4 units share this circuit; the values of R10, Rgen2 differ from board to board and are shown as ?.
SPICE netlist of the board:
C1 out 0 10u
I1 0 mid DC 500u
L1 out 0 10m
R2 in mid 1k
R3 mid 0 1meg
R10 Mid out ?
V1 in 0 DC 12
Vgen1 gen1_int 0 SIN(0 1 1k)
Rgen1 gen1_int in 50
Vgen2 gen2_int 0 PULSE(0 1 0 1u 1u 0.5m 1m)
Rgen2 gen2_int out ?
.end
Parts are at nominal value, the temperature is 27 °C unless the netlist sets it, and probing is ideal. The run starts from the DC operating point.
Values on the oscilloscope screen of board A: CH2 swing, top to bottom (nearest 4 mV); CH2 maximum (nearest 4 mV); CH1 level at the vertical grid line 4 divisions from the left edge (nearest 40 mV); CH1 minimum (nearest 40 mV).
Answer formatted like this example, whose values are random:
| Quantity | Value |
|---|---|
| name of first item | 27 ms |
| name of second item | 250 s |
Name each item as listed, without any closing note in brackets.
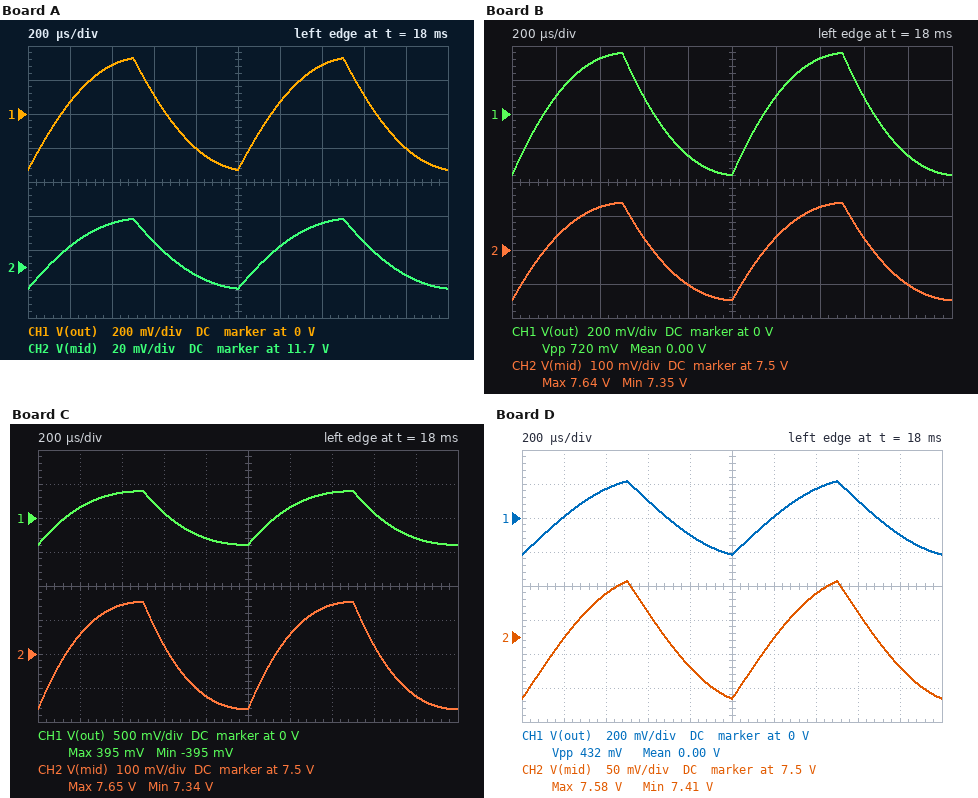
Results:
| Quantity | Value |
|---|---|
| CH2 swing, top to bottom | 40 mV |
| CH2 maximum | 11.728 V |
| CH1 level at the vertical grid line 4 divisions from the left edge | -200 mV |
| CH1 minimum | -320 mV |
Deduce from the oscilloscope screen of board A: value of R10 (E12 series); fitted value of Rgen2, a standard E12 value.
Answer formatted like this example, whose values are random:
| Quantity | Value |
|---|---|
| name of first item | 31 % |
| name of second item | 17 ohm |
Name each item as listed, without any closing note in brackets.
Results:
| Quantity | Value |
|---|---|
| value of R10 | 15 kΩ |
| fitted value of Rgen2, a standard E12 value | 39 Ω |
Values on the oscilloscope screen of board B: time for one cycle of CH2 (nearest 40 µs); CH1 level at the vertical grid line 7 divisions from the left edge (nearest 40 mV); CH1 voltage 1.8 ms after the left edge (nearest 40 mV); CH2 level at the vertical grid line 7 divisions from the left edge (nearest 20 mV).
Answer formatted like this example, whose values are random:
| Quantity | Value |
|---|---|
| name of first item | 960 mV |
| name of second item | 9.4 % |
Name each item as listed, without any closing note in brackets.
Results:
| Quantity | Value |
|---|---|
| time for one cycle of CH2 | 1.00 ms |
| CH1 level at the vertical grid line 7 divisions from the left edge | 320 mV |
| CH1 voltage 1.8 ms after the left edge | -240 mV |
| CH2 level at the vertical grid line 7 divisions from the left edge | 7.62 V |
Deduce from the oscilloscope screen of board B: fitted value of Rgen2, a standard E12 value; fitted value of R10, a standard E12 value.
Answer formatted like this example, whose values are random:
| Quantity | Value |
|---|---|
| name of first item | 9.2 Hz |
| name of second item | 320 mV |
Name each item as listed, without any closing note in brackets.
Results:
| Quantity | Value |
|---|---|
| fitted value of Rgen2, a standard E12 value | 33 Ω |
| fitted value of R10, a standard E12 value | 1.5 kΩ |
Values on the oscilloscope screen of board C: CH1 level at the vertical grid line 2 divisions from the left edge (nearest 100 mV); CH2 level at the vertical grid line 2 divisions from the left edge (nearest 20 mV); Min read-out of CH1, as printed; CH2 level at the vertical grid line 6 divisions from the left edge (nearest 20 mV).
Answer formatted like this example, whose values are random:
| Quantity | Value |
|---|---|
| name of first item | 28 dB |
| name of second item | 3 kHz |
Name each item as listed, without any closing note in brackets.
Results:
| Quantity | Value |
|---|---|
| CH1 level at the vertical grid line 2 divisions from the left edge | 400 mV |
| CH2 level at the vertical grid line 2 divisions from the left edge | 7.64 V |
| Min read-out of CH1, as printed | -395 mV |
| CH2 level at the vertical grid line 6 divisions from the left edge | 7.56 V |
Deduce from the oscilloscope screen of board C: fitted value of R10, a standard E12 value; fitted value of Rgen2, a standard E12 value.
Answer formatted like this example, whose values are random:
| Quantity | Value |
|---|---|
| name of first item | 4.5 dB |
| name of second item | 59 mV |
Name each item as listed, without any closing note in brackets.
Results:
| Quantity | Value |
|---|---|
| fitted value of R10, a standard E12 value | 1.5 kΩ |
| fitted value of Rgen2, a standard E12 value | 27 Ω |
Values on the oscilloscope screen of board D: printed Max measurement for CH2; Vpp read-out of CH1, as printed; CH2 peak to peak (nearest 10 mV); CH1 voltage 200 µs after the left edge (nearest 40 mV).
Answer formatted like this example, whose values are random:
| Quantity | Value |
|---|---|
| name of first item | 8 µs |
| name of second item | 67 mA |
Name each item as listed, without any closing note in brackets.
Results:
| Quantity | Value |
|---|---|
| printed Max measurement for CH2 | 7.58 V |
| Vpp read-out of CH1, as printed | 432 mV |
| CH2 peak to peak | 170 mV |
| CH1 voltage 200 µs after the left edge | 0 V |
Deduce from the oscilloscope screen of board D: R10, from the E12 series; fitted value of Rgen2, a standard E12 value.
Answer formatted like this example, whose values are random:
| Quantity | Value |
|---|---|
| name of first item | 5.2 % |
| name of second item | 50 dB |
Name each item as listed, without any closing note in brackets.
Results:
| Quantity | Value |
|---|---|
| R10, from the E12 series | 1.5 kΩ |
| fitted value of Rgen2, a standard E12 value | 68 Ω |
